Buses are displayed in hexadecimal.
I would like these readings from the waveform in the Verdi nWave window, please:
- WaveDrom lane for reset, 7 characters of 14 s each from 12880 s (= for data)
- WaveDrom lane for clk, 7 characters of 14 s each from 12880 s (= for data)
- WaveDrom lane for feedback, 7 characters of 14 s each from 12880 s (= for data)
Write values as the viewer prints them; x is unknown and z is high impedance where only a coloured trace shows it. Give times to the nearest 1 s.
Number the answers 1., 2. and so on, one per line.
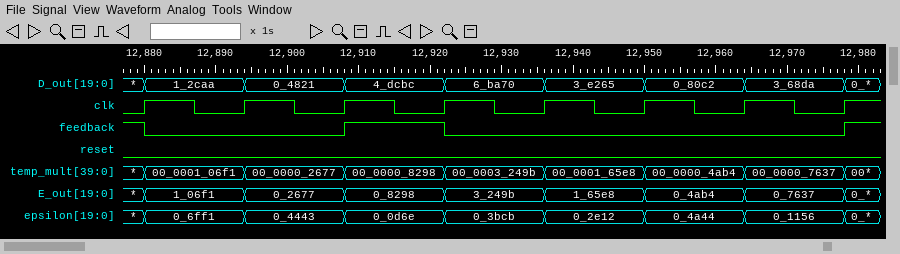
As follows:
1. {name: 'reset', wave: '0......'}
2. {name: 'clk', wave: 'p......'}
3. {name: 'feedback', wave: '0.10...'}
